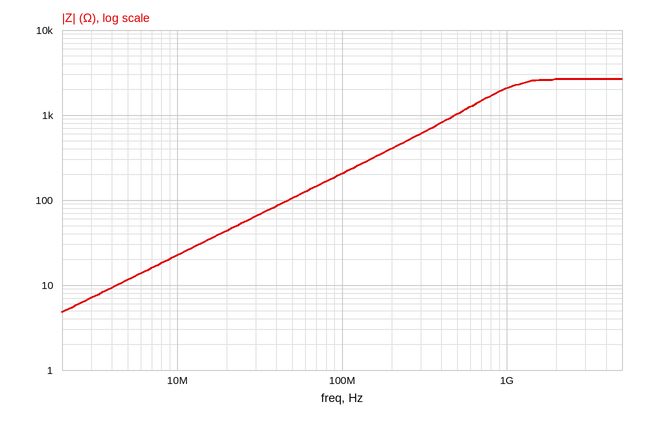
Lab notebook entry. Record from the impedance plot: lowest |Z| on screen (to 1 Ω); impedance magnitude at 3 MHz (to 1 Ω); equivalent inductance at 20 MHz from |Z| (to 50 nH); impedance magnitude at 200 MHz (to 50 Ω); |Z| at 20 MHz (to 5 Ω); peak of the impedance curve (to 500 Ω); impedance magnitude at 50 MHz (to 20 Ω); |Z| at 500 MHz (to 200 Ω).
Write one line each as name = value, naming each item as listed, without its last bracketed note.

lowest |Z| on screen = 5 Ω
impedance magnitude at 3 MHz = 7 Ω
equivalent inductance at 20 MHz from |Z| = 350 nH
impedance magnitude at 200 MHz = 400 Ω
|Z| at 20 MHz = 45 Ω
peak of the impedance curve = 2.5 kΩ
impedance magnitude at 50 MHz = 100 Ω
|Z| at 500 MHz = 1.0 kΩ
